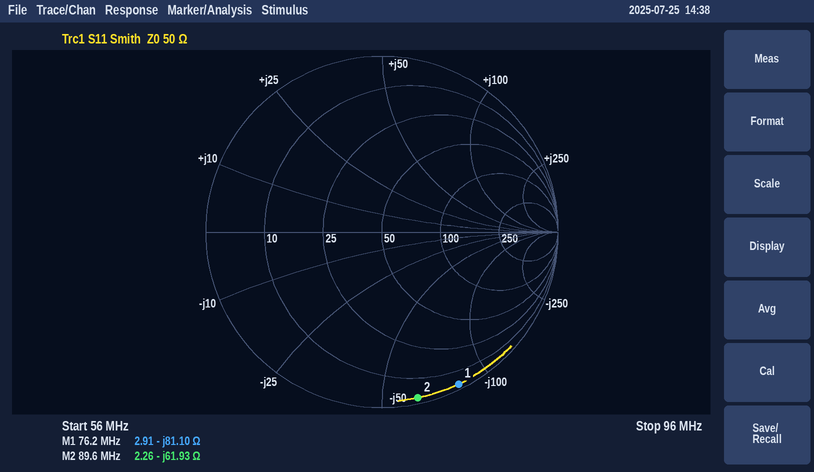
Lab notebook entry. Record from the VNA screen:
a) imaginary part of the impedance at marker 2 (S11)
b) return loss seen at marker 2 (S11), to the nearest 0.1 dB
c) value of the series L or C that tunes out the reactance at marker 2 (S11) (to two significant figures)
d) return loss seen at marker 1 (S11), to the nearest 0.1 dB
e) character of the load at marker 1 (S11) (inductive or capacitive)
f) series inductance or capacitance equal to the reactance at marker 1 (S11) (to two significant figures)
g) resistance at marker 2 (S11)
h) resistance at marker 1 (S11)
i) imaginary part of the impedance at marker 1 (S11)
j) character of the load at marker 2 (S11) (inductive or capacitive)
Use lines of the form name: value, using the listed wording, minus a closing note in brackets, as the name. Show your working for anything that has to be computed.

imaginary part of the impedance at marker 2: -61.93 Ω
return loss seen at marker 2 (S11), to the nearest 0.1 dB: 0.3 dB
value of the series L or C that tunes out the reactance at marker 2 (S11): L = 61.93 Ω/(2π × 89.6 MHz) ≈ 110 nH
return loss seen at marker 1 (S11), to the nearest 0.1 dB: 0.3 dB
character of the load at marker 1 (S11): capacitive
series inductance or capacitance equal to the reactance at marker 1 (S11): C = 1/(2π × 76.2 MHz × 81.1 Ω) ≈ 26 pF
resistance at marker 2: 2.26 Ω
resistance at marker 1: 2.91 Ω
imaginary part of the impedance at marker 1: -81.10 Ω
character of the load at marker 2 (S11): capacitive
